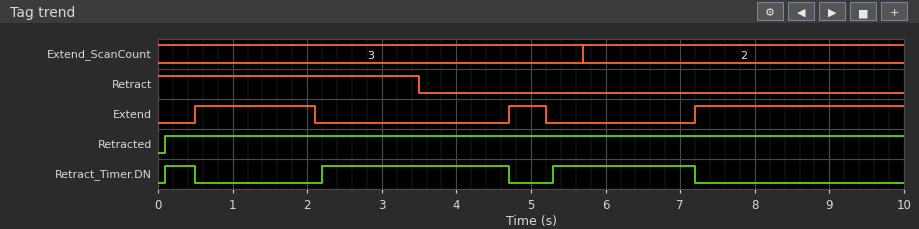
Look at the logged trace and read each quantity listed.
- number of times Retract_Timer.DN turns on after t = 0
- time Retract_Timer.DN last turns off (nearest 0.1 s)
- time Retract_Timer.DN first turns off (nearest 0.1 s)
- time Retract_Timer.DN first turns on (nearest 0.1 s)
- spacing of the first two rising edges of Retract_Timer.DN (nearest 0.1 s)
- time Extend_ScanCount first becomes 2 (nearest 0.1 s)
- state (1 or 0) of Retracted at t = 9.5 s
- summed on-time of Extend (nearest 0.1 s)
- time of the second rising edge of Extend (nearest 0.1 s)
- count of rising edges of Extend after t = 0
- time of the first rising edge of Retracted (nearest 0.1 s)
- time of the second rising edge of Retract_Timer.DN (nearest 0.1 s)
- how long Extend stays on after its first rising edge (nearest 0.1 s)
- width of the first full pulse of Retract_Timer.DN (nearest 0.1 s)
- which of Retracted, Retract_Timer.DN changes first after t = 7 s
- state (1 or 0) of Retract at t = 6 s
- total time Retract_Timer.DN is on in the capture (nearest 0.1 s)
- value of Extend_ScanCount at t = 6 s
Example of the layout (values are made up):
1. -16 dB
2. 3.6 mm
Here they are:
1. 3
2. 7.2 s
3. 0.5 s
4. 0.1 s
5. 2.1 s
6. 5.7 s
7. 1
8. 4.9 s
9. 4.7 s
10. 3
11. 0.1 s
12. 2.2 s
13. 1.6 s
14. 0.4 s
15. Retract_Timer.DN
16. 0
17. 4.8 s
18. 2
